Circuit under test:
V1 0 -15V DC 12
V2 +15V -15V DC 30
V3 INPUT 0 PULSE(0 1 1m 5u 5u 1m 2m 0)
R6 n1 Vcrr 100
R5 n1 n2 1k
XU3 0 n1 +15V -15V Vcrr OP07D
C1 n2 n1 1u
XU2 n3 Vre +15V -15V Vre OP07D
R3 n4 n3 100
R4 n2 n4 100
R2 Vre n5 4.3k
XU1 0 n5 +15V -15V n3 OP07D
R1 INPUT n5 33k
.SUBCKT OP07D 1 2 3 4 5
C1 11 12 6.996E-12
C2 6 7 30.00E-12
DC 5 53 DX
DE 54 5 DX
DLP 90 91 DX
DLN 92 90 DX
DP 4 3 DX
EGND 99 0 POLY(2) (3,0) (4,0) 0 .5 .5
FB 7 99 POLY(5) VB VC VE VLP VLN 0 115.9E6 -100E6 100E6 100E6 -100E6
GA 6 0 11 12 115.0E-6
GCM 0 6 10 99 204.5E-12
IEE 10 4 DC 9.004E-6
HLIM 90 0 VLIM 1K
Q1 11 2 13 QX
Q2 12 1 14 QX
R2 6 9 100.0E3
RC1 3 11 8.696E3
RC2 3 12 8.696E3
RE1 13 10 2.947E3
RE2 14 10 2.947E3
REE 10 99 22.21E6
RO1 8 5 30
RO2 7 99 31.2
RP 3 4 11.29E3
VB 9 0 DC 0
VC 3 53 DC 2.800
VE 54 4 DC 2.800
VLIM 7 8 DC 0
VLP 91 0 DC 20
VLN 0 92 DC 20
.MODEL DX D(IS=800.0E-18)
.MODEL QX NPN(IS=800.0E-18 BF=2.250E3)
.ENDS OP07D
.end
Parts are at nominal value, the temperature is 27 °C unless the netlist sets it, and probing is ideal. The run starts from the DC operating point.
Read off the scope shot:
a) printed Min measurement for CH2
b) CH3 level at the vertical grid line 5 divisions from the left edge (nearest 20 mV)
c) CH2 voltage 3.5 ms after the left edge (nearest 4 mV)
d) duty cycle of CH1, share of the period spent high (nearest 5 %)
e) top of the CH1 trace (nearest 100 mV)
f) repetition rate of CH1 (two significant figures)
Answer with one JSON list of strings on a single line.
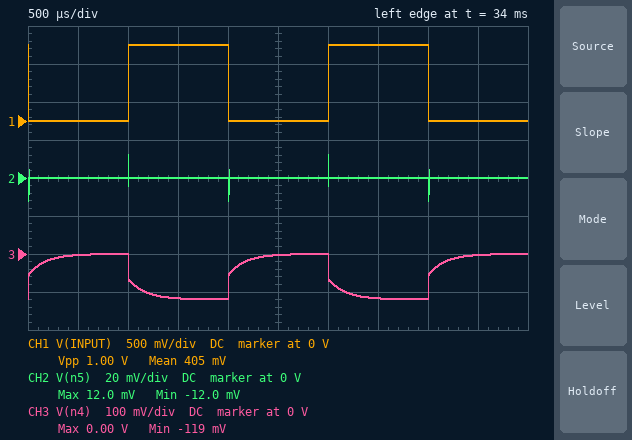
["-12.0 mV", "0 V", "0 V", "50 %", "1.0 V", "500 Hz"]
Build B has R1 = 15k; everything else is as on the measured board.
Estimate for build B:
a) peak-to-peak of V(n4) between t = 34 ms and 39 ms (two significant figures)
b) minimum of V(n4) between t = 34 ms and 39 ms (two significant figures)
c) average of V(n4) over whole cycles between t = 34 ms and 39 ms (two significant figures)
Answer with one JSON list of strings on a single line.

["260 mV", "-260 mV", "-130 mV"]
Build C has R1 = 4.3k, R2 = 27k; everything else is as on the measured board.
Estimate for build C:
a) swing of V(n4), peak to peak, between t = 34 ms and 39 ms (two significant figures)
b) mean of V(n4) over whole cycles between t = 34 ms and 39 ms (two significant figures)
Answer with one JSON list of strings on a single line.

["5.7 V", "-2.9 V"]
